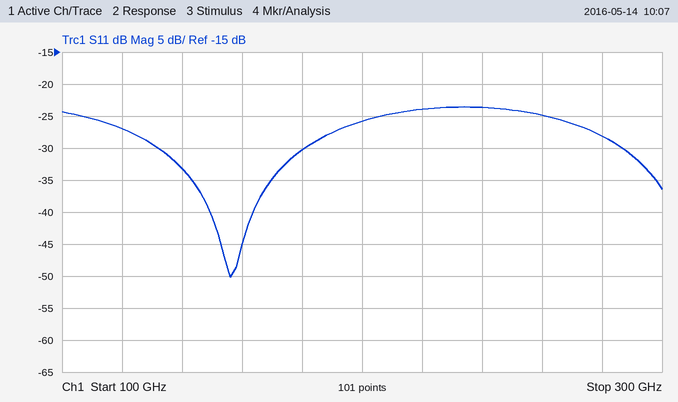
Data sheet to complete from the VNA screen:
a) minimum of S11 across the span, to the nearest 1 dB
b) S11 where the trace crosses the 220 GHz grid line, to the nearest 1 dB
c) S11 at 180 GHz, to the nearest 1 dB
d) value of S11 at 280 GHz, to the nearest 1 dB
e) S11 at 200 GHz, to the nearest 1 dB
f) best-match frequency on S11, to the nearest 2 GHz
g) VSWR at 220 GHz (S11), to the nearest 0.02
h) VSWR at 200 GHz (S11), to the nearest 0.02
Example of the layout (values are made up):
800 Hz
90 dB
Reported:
-50 dB
-24 dB
-30 dB
-28 dB
-26 dB
156 GHz
1.14
1.10
